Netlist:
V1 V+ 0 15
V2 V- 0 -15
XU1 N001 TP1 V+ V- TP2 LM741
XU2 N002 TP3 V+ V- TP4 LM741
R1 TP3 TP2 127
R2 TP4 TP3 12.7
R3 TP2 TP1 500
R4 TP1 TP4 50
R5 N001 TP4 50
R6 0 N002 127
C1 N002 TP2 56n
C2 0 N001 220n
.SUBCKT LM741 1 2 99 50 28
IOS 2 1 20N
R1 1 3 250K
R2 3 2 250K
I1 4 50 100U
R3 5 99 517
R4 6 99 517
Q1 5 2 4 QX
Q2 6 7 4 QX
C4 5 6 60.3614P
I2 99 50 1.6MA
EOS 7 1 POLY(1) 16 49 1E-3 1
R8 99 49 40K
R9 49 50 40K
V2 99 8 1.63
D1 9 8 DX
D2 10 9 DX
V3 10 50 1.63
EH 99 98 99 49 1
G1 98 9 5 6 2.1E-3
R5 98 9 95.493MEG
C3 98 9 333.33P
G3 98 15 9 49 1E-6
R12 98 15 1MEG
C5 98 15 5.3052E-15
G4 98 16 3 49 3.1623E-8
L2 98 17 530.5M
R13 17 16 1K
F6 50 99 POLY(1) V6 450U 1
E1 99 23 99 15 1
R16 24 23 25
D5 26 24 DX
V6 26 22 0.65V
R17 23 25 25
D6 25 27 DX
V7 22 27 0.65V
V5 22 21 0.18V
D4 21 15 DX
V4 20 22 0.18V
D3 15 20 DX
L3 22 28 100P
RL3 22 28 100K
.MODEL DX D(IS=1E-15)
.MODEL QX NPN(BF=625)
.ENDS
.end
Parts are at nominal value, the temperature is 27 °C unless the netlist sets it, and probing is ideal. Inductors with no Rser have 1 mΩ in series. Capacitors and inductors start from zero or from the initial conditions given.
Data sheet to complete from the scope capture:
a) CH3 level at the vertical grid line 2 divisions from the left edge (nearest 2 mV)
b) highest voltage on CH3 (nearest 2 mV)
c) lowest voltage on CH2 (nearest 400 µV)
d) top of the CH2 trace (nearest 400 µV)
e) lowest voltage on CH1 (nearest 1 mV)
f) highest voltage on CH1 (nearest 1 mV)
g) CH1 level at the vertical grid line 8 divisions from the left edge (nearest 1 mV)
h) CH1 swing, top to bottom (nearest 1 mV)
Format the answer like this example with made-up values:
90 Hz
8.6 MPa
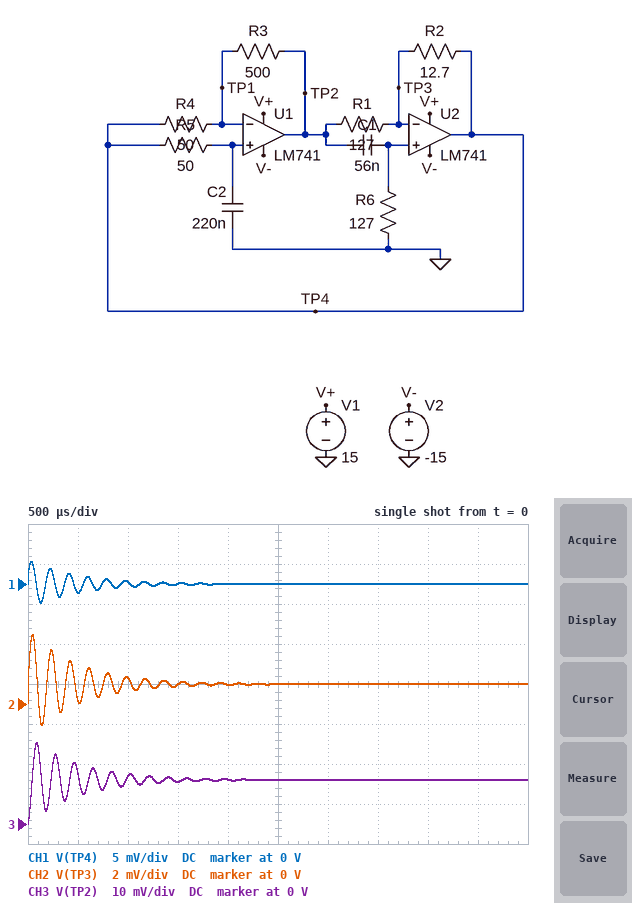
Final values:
12 mV
20 mV
-1.2 mV
3.6 mV
-2 mV
3 mV
0 V
5 mV
